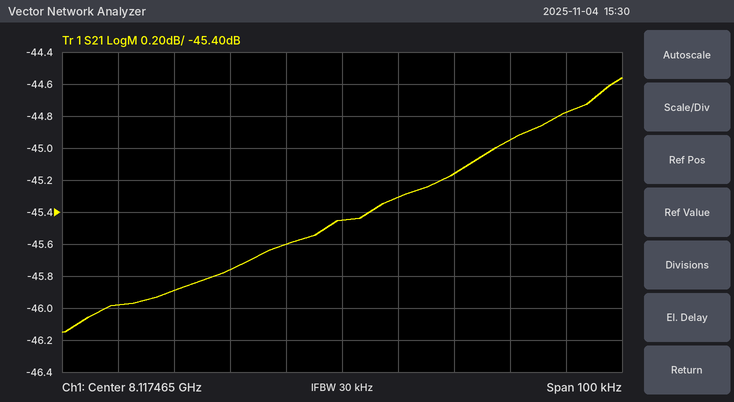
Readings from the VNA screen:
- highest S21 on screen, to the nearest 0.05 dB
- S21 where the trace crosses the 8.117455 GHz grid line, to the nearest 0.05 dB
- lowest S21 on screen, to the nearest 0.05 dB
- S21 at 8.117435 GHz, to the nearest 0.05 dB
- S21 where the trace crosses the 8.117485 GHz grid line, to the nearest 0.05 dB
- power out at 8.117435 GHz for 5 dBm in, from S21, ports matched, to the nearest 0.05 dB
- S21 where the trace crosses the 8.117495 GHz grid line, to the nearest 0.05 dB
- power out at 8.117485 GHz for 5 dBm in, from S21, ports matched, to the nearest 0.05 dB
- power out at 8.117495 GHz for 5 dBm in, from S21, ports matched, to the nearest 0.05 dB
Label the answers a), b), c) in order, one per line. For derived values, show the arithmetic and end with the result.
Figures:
a) -44.55 dB
b) -45.60 dB
c) -46.15 dB
d) -45.90 dB
e) -45.15 dB
f) 5 dBm + (-45.90 dB) = -40.90 dBm
g) -44.95 dB
h) 5 dBm + (-45.15 dB) = -40.15 dBm
i) 5 dBm + (-44.95 dB) = -39.95 dBm
